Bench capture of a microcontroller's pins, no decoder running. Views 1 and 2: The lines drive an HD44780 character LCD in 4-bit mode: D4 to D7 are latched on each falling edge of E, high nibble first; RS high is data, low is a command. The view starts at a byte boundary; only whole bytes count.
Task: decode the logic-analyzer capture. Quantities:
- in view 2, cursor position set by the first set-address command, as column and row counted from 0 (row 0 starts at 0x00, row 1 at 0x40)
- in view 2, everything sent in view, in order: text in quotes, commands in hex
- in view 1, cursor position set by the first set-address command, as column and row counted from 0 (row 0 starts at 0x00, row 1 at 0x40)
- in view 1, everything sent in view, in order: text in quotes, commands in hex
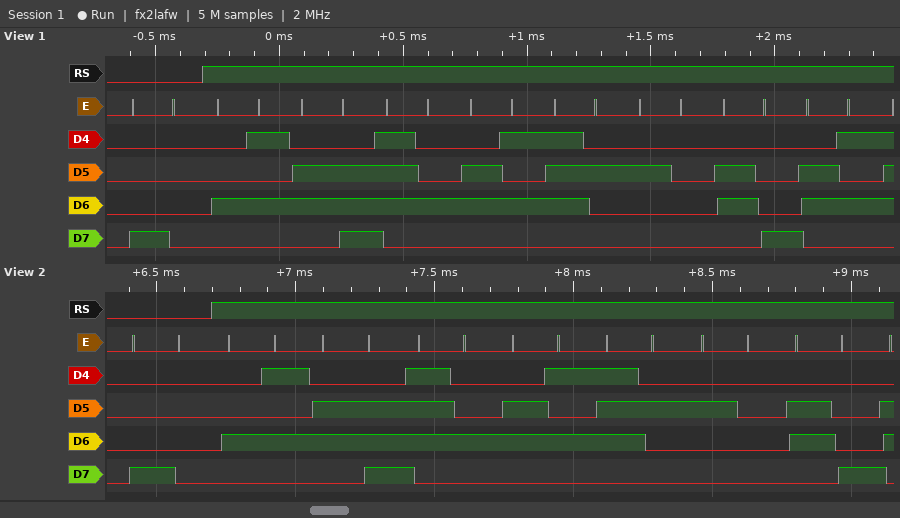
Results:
column 0, row 0
0x80 "Enter h"
column 0, row 0
0x80 "Enter he"
